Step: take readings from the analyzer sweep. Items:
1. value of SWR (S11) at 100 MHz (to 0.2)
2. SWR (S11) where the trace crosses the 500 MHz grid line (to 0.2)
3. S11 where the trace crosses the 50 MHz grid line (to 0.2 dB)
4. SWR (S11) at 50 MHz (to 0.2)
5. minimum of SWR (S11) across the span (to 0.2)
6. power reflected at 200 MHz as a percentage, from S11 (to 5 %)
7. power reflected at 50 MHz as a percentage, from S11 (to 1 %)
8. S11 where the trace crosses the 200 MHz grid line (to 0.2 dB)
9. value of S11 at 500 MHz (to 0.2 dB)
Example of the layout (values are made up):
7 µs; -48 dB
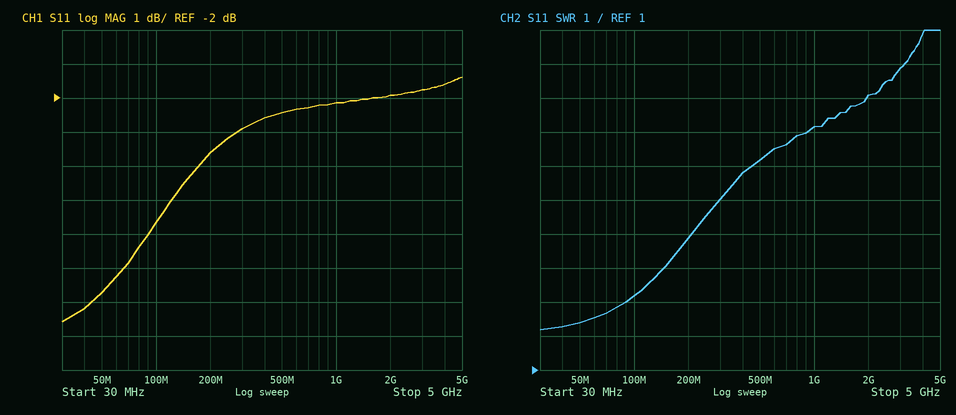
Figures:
3.2; 7.2; -7.8 dB; 2.4; 2.2; 45 %; 17 %; -3.6 dB; -2.4 dB
